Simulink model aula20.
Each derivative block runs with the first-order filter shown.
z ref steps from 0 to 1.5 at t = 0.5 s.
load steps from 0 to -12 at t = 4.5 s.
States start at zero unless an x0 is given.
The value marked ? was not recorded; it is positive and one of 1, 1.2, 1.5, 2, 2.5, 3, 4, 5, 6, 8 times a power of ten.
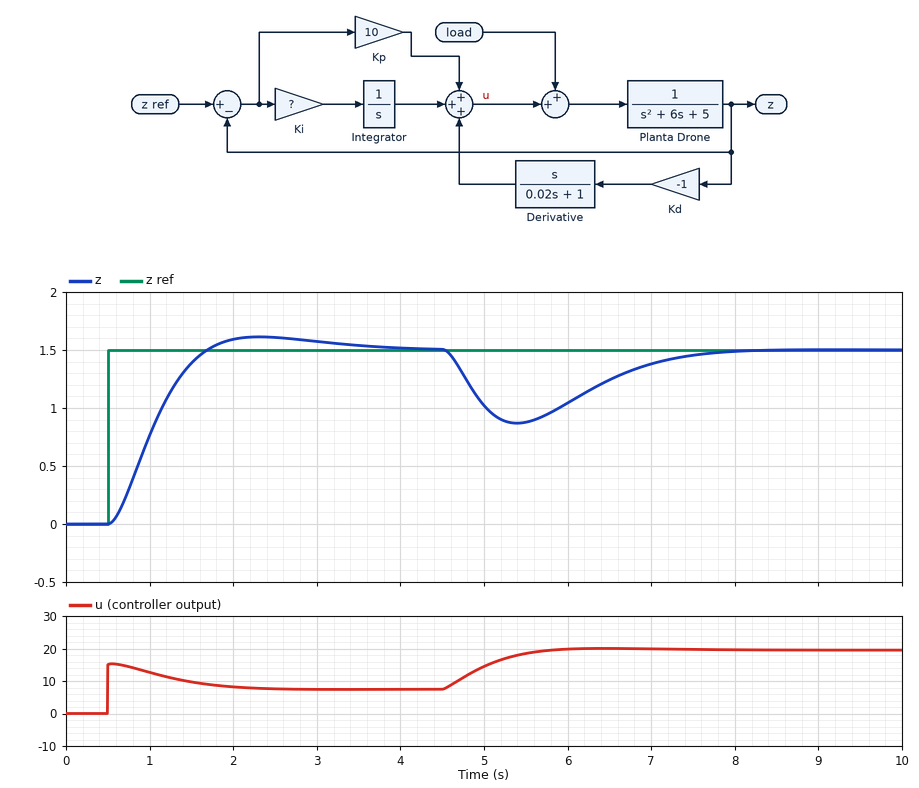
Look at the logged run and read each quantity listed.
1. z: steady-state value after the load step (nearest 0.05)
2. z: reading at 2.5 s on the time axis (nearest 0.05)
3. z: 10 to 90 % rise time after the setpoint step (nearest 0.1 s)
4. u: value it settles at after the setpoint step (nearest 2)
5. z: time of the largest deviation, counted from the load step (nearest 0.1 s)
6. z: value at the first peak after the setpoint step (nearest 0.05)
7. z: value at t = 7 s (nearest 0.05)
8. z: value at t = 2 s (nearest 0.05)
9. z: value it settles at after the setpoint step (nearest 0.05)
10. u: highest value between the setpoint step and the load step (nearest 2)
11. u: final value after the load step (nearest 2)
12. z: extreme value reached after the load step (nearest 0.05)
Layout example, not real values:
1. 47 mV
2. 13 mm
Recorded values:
1. 1.50
2. 1.60
3. 0.8 s
4. 8
5. 0.9 s
6. 1.60
7. 1.40
8. 1.60
9. 1.50
10. 16
11. 20
12. 0.85
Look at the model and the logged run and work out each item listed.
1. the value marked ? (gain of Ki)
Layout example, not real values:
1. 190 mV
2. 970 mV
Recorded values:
1. 12
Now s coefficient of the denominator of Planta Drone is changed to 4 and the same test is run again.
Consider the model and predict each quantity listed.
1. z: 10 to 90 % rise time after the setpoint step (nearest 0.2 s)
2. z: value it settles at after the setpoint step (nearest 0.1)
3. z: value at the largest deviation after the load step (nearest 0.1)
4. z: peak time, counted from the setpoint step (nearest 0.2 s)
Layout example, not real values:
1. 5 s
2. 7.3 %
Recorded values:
1. 0.6 s
2. 1.5
3. 0.8
4. 1.2 s
